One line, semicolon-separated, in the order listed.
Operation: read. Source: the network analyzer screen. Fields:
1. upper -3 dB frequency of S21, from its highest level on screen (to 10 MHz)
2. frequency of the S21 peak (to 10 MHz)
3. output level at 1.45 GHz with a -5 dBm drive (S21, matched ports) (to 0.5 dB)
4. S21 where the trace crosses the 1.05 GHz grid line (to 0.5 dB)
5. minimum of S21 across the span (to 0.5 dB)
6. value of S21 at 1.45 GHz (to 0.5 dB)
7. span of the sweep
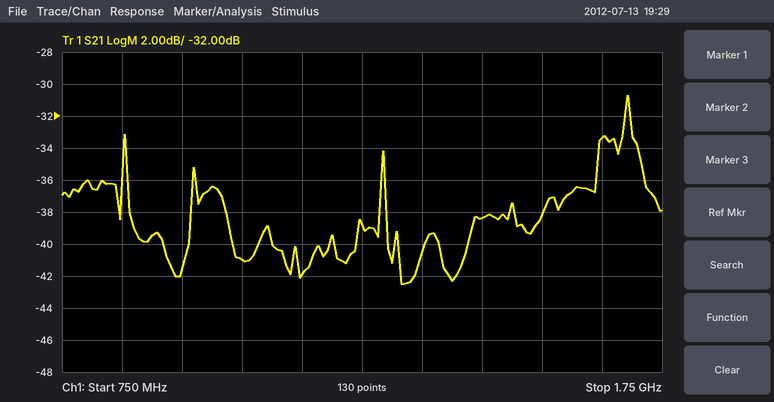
1.71 GHz; 1.69 GHz; -43.5 dBm; -41.0 dB; -42.5 dB; -38.5 dB; 1 GHz
